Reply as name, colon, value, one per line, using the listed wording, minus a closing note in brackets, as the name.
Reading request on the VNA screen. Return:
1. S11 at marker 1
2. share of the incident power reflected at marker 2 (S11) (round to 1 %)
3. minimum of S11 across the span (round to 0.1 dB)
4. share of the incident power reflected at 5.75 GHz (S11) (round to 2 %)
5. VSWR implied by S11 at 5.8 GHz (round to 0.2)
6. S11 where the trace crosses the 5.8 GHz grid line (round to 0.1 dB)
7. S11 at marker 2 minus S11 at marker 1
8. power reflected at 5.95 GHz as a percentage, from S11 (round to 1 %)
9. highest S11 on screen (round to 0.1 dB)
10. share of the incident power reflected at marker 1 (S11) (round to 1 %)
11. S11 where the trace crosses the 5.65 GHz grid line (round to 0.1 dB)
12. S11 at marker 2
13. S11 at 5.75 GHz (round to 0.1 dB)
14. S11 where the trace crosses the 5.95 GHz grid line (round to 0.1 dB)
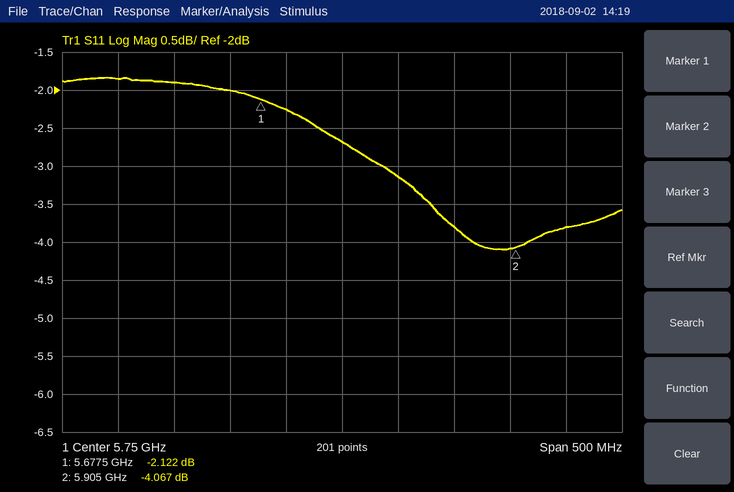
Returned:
S11 at marker 1: -2.122 dB
share of the incident power reflected at marker 2 (S11): 39 %
minimum of S11 across the span: -4.1 dB
share of the incident power reflected at 5.75 GHz (S11): 54 %
VSWR implied by S11 at 5.8 GHz: 5.6
S11 where the trace crosses the 5.8 GHz grid line: -3.1 dB
S11 at marker 2 minus S11 at marker 1: -1.945 dB
power reflected at 5.95 GHz as a percentage, from S11: 42 %
highest S11 on screen: -1.8 dB
share of the incident power reflected at marker 1 (S11): 61 %
S11 where the trace crosses the 5.65 GHz grid line: -2.0 dB
S11 at marker 2: -4.067 dB
S11 at 5.75 GHz: -2.7 dB
S11 where the trace crosses the 5.95 GHz grid line: -3.8 dB
